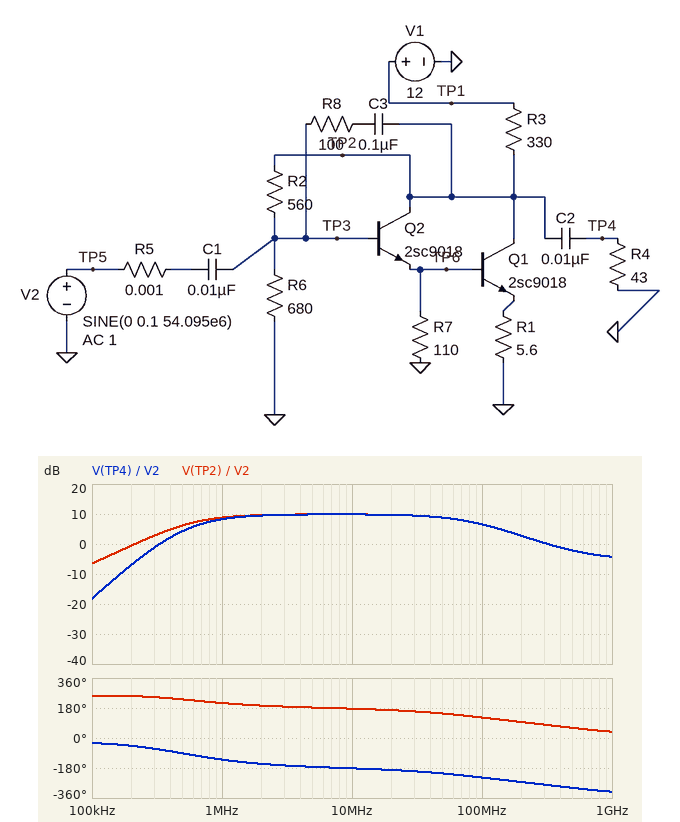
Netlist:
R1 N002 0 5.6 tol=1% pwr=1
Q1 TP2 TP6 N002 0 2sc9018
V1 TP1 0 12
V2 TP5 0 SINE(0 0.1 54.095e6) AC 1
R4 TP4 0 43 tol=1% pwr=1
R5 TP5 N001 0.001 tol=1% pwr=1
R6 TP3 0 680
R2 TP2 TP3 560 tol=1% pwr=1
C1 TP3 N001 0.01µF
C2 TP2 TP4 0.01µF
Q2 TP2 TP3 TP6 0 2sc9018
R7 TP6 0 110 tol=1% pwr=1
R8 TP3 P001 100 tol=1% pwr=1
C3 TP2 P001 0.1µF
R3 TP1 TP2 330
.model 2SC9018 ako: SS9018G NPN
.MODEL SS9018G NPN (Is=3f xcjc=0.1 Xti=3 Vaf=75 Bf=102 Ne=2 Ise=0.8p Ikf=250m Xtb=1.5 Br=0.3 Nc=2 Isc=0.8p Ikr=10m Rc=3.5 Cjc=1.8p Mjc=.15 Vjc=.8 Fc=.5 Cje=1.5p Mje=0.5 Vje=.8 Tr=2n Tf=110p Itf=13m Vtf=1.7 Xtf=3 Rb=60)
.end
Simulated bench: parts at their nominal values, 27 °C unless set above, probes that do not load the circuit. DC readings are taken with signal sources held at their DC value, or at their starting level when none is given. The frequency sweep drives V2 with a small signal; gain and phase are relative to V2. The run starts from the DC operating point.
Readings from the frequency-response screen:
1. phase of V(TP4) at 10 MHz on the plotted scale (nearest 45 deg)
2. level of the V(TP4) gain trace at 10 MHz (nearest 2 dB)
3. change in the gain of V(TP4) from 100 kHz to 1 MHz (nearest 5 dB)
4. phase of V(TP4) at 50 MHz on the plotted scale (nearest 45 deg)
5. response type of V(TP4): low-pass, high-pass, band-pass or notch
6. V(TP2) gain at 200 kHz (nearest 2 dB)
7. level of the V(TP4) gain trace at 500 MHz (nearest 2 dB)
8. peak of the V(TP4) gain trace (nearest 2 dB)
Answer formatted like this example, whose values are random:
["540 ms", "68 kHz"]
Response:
["-180 deg", "10 dB", "25 dB", "-225 deg", "band-pass", "0 dB", "-2 dB", "10 dB"]
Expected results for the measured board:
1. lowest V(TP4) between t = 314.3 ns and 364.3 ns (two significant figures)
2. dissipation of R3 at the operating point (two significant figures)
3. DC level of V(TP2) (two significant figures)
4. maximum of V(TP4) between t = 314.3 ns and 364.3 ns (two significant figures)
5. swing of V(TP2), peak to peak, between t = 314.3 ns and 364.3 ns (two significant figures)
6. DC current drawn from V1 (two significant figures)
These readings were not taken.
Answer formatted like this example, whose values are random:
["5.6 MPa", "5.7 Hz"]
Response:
["-260 mV", "250 mW", "3.0 V", "270 mV", "530 mV", "27 mA"]
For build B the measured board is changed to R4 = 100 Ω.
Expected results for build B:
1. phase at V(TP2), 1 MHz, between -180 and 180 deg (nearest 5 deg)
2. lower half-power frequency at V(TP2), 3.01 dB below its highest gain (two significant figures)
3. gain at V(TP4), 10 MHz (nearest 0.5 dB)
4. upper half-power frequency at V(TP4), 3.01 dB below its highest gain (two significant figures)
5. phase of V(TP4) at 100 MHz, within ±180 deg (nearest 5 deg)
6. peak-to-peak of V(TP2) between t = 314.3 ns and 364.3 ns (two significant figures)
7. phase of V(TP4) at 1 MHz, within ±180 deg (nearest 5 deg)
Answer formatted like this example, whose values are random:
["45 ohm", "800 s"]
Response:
["-135 deg", "1.0 MHz", "13.5 dB", "90 MHz", "120 deg", "800 mV", "-125 deg"]
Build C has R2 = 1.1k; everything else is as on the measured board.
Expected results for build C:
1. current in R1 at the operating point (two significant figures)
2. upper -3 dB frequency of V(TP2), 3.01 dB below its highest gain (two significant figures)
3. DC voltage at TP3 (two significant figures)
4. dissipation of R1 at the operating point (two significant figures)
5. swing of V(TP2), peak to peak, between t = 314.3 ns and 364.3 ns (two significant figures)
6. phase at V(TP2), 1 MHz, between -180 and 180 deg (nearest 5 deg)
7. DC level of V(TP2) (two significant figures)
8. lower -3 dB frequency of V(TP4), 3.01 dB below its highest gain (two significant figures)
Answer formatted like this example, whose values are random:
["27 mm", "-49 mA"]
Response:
["14 mA", "130 MHz", "1.6 V", "1.0 mW", "540 mV", "-155 deg", "4.2 V", "660 kHz"]
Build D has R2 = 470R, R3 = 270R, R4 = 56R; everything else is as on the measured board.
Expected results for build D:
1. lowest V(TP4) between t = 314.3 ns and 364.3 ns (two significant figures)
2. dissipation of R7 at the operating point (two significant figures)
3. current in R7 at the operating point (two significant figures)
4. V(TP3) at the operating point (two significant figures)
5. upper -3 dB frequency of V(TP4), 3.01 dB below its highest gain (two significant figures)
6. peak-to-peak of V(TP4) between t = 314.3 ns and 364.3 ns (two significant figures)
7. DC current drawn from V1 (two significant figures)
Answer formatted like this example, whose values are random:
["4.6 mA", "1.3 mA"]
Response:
["-290 mV", "7.6 mW", "8.3 mA", "1.7 V", "75 MHz", "600 mV", "34 mA"]
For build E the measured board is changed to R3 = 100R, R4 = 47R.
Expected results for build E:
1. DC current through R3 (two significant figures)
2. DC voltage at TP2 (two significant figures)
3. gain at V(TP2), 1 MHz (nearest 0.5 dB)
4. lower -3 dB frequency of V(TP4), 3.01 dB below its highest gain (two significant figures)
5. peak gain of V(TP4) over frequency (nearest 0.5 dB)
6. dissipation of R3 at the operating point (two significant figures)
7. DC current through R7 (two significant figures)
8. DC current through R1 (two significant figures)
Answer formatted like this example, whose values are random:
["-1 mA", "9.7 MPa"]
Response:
["83 mA", "3.7 V", "8.5 dB", "760 kHz", "10.0 dB", "690 mW", "11 mA", "69 mA"]
